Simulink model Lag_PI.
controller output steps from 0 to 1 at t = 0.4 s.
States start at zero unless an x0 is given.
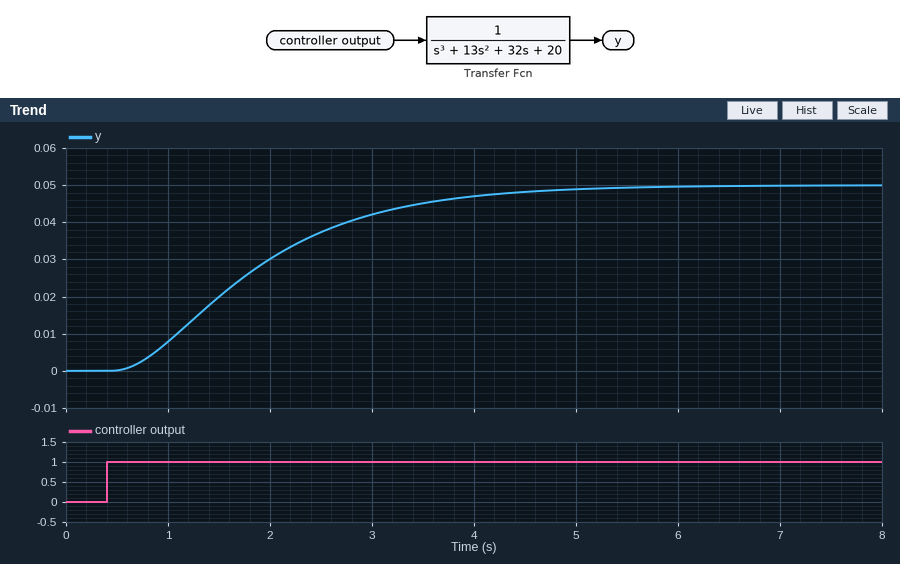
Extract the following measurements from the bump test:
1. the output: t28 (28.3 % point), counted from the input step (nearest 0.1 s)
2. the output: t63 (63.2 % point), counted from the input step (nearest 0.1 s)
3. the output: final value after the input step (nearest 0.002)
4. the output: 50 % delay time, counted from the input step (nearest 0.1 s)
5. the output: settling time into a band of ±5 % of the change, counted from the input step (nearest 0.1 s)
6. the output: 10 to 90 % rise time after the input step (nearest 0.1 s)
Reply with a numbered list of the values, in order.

1. 0.9 s
2. 1.7 s
3. 0.050
4. 1.3 s
5. 3.8 s
6. 2.6 s
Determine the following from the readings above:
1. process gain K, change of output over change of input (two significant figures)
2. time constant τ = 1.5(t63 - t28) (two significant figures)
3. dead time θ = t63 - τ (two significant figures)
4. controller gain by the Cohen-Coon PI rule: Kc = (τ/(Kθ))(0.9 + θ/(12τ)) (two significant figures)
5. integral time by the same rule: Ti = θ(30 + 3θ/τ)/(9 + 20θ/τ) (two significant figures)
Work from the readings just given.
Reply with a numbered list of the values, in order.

1. 0.050
2. 1.2 s
3. 0.50 s
4. 45
5. 0.90 s
